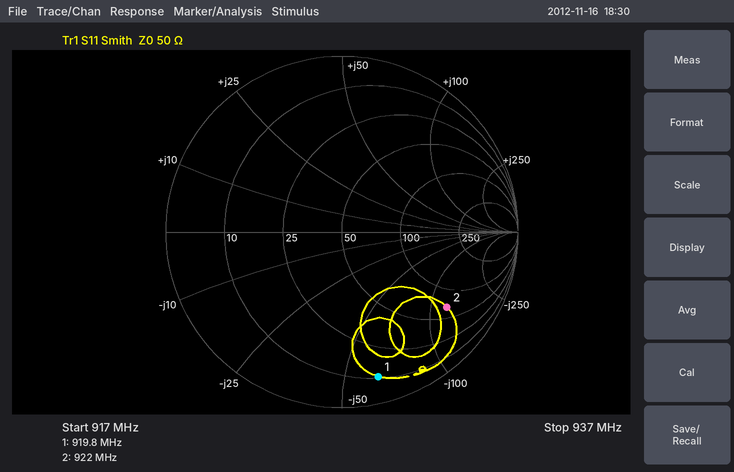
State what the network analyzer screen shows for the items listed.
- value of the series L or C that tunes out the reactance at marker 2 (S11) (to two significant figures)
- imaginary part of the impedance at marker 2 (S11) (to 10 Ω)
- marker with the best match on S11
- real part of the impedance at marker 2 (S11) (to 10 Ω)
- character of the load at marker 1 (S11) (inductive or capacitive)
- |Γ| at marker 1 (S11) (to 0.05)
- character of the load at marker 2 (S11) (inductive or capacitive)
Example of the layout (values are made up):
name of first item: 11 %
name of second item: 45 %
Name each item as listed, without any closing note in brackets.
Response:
value of the series L or C that tunes out the reactance at marker 2 (S11): 21 nH
imaginary part of the impedance at marker 2 (S11): -120 Ω
marker with the best match on S11: marker 2
real part of the impedance at marker 2 (S11): 70 Ω
character of the load at marker 1 (S11): capacitive
|Γ| at marker 1 (S11): 0.85
character of the load at marker 2 (S11): capacitive
